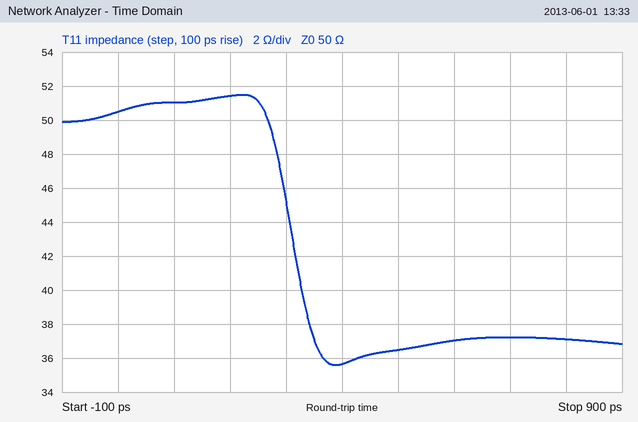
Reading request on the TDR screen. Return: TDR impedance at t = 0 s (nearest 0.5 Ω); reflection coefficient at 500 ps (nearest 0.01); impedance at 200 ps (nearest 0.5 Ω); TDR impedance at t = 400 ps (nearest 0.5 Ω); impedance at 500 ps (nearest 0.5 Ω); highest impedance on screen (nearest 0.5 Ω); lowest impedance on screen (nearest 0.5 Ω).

50.5 Ω
-0.16
51.5 Ω
35.5 Ω
36.5 Ω
51.5 Ω
35.5 Ω
